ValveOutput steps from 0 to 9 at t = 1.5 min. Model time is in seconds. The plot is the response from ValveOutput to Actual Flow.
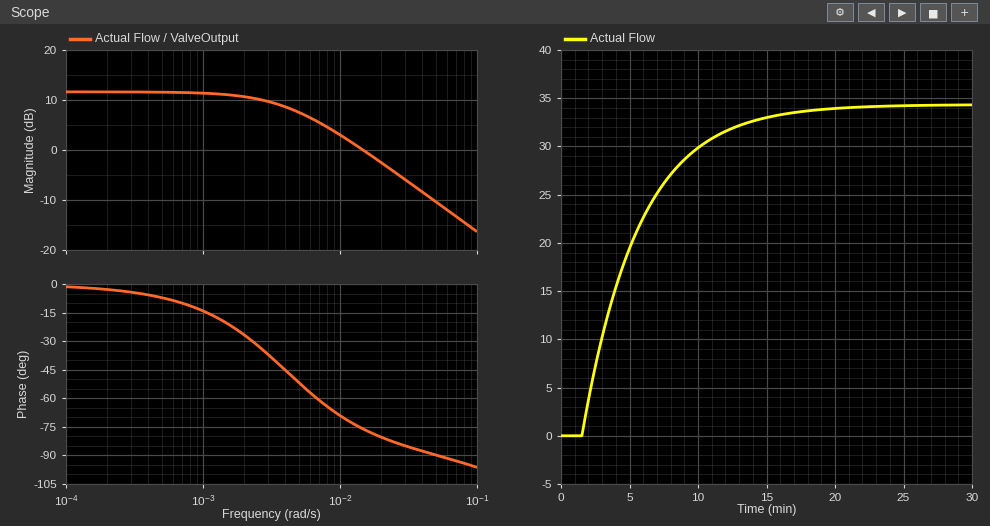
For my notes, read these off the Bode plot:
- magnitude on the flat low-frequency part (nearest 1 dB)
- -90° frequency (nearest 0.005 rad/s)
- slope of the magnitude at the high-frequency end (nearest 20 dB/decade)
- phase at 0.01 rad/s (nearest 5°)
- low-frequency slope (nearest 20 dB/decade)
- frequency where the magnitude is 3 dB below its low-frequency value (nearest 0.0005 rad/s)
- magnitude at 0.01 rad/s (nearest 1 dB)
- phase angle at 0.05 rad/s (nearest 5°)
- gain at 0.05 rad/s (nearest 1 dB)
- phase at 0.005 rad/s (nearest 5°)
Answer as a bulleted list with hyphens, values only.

- 12 dB
- 0.050 rad/s
- -20 dB/decade
- -70°
- 0 dB/decade
- 0.0040 rad/s
- 3 dB
- -90°
- -10 dB
- -50°
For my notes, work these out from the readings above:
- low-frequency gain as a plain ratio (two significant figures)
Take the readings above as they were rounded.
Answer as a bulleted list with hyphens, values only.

- 4.0
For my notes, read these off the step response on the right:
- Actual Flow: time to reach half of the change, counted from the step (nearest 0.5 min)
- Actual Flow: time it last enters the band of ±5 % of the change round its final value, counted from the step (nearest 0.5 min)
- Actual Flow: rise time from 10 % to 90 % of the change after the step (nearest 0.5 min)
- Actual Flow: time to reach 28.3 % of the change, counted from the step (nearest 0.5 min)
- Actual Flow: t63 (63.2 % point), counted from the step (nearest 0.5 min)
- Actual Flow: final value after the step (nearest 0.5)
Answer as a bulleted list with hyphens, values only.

- 3.0 min
- 12.5 min
- 9.0 min
- 1.5 min
- 4.0 min
- 34.5
